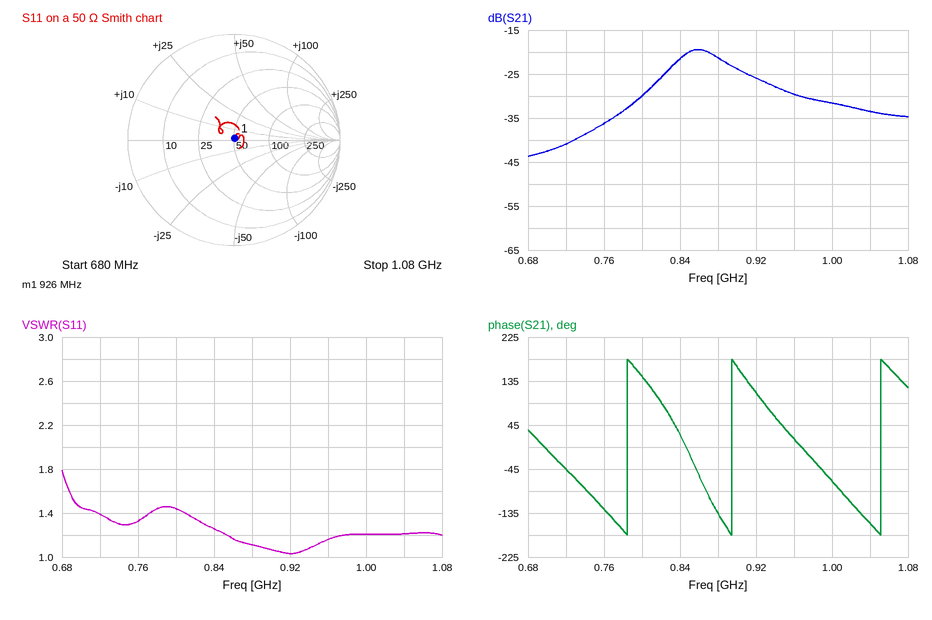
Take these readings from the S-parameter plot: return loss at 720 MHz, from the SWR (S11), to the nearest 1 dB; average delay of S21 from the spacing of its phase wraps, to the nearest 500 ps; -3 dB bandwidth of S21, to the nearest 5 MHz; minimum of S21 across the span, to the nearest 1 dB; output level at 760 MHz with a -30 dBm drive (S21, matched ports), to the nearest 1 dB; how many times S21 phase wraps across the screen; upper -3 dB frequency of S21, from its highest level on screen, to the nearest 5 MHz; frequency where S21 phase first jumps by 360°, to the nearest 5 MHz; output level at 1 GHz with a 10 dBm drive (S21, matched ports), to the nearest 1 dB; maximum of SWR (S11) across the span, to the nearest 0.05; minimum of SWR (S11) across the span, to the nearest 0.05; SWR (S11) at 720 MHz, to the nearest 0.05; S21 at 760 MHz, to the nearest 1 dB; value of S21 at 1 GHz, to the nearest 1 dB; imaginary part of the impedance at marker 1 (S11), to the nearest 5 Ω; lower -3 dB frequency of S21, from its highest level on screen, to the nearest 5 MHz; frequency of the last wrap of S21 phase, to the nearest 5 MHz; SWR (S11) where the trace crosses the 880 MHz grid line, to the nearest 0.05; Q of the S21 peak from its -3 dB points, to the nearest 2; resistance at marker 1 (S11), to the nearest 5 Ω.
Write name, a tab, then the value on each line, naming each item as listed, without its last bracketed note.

return loss at 720 MHz, from the SWR (S11), to the nearest 1 dB	16 dB
average delay of S21 from the spacing of its phase wraps, to the nearest 500 ps	7.5 ns
-3 dB bandwidth of S21, to the nearest 5 MHz	55 MHz
minimum of S21 across the span, to the nearest 1 dB	-44 dB
output level at 760 MHz with a -30 dBm drive (S21, matched ports), to the nearest 1 dB	-66 dBm
how many times S21 phase wraps across the screen	3
upper -3 dB frequency of S21, from its highest level on screen, to the nearest 5 MHz	890 MHz
frequency where S21 phase first jumps by 360°, to the nearest 5 MHz	785 MHz
output level at 1 GHz with a 10 dBm drive (S21, matched ports), to the nearest 1 dB	-22 dBm
maximum of SWR (S11) across the span, to the nearest 0.05	1.80
minimum of SWR (S11) across the span, to the nearest 0.05	1.05
SWR (S11) at 720 MHz, to the nearest 0.05	1.40
S21 at 760 MHz, to the nearest 1 dB	-36 dB
value of S21 at 1 GHz, to the nearest 1 dB	-32 dB
imaginary part of the impedance at marker 1 (S11), to the nearest 5 Ω	0 Ω
lower -3 dB frequency of S21, from its highest level on screen, to the nearest 5 MHz	835 MHz
frequency of the last wrap of S21 phase, to the nearest 5 MHz	1.050 GHz
SWR (S11) where the trace crosses the 880 MHz grid line, to the nearest 0.05	1.10
Q of the S21 peak from its -3 dB points, to the nearest 2	16
resistance at marker 1 (S11), to the nearest 5 Ω	50 Ω
